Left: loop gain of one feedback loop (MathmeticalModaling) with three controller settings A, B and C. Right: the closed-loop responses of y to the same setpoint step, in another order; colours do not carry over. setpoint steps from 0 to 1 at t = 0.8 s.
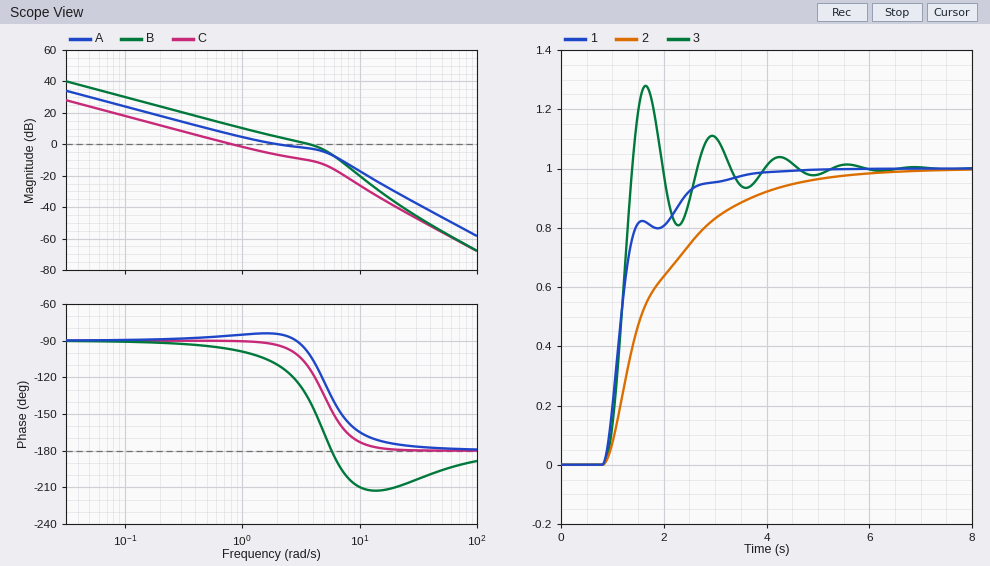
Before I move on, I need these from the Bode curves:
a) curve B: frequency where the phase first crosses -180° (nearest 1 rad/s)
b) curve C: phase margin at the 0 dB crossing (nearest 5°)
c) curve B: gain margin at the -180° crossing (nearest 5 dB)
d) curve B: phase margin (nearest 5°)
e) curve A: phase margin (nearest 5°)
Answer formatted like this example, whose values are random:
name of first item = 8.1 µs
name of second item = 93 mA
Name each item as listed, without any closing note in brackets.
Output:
curve B: frequency where the phase first crosses -180° = 6 rad/s
curve C: phase margin at the 0 dB crossing = 90°
curve B: gain margin at the -180° crossing = 5 dB
curve B: phase margin = 40°
curve A: phase margin = 95°
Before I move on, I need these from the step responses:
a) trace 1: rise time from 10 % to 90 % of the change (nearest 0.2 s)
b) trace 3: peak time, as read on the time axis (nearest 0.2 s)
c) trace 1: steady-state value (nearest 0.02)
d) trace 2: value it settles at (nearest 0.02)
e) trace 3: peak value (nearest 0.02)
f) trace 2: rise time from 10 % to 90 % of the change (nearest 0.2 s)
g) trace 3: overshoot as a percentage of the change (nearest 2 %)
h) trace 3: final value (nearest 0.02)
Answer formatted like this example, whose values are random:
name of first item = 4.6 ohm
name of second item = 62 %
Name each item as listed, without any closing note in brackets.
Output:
trace 1: rise time from 10 % to 90 % of the change = 1.4 s
trace 3: peak time, as read on the time axis = 1.6 s
trace 1: steady-state value = 1.00
trace 2: value it settles at = 1.00
trace 3: peak value = 1.28
trace 2: rise time from 10 % to 90 % of the change = 2.6 s
trace 3: overshoot as a percentage of the change = 28 %
trace 3: final value = 1.00
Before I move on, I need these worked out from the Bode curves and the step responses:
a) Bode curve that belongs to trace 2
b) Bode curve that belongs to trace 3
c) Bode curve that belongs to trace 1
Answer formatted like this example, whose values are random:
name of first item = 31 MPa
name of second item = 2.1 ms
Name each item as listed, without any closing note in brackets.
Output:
Bode curve that belongs to trace 2 = C
Bode curve that belongs to trace 3 = B
Bode curve that belongs to trace 1 = A
